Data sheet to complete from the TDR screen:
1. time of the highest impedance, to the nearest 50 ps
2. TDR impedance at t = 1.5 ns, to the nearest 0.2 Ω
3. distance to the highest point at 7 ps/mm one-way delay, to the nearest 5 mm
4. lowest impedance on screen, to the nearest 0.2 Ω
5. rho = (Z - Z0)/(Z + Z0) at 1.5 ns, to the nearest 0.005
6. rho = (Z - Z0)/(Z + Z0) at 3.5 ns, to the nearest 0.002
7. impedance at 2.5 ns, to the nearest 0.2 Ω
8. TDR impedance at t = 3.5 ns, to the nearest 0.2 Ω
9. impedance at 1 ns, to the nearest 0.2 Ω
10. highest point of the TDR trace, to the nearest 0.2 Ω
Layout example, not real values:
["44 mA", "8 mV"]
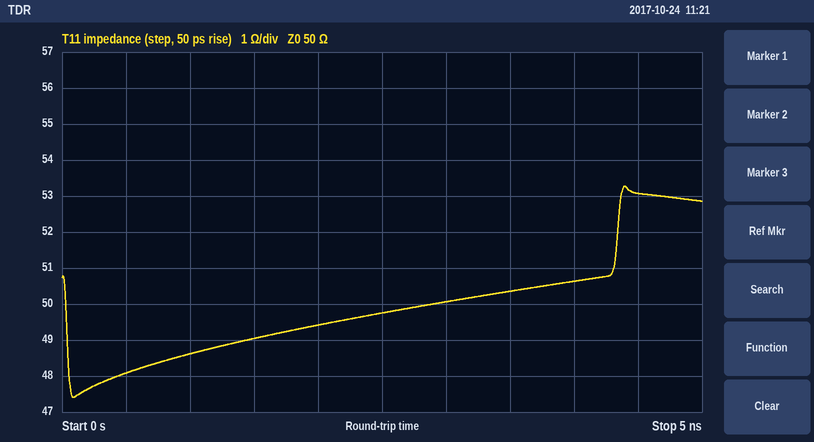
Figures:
["4.40 ns", "49.0 Ω", "315 mm", "47.4 Ω", "-0.010", "+0.004", "49.8 Ω", "50.4 Ω", "48.6 Ω", "53.2 Ω"]
